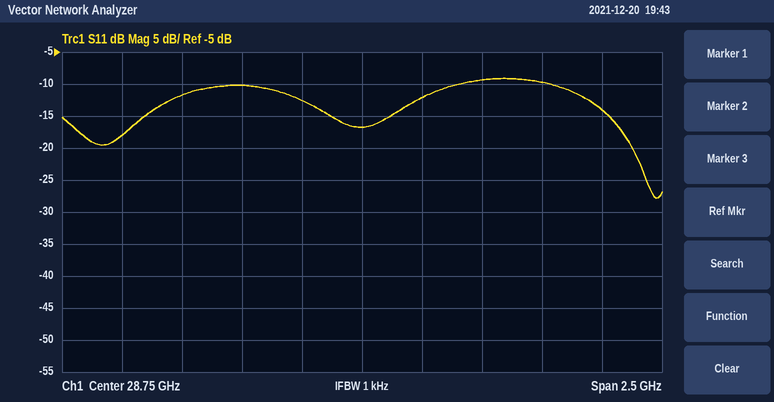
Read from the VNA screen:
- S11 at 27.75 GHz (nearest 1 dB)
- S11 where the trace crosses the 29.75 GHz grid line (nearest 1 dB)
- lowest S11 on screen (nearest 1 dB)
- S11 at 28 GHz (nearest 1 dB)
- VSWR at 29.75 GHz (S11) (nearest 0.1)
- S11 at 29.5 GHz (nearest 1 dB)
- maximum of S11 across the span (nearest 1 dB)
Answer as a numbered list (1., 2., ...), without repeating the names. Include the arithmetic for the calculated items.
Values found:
1. -18 dB
2. -14 dB
3. -28 dB
4. -12 dB
5. |Γ| = 10^(-14/20) = 0.1995; VSWR = (1 + 0.1995)/(1 − 0.1995) ≈ 1.5
6. -10 dB
7. -9 dB
